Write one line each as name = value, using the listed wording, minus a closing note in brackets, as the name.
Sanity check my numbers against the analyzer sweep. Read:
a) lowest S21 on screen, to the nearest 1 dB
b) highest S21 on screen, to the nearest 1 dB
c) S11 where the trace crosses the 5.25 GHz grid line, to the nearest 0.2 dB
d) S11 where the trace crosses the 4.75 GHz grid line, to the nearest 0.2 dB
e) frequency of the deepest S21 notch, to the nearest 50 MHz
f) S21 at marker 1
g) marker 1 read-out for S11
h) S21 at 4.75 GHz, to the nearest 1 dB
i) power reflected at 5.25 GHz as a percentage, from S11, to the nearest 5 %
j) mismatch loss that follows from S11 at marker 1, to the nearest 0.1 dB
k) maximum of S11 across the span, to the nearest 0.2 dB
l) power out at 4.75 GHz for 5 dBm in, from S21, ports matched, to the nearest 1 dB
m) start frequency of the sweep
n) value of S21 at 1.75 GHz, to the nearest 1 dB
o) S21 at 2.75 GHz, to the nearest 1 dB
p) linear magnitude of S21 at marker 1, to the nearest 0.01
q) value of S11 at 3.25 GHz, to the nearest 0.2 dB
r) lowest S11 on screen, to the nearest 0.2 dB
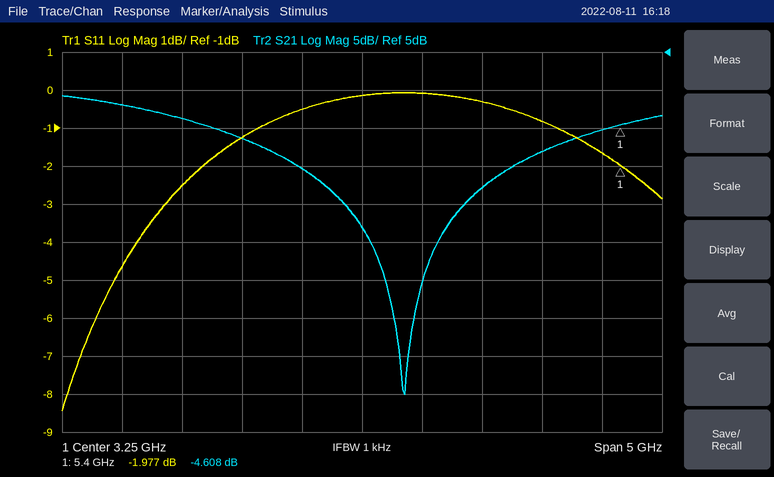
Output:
lowest S21 on screen, to the nearest 1 dB = -40 dB
highest S21 on screen, to the nearest 1 dB = -1 dB
S11 where the trace crosses the 5.25 GHz grid line, to the nearest 0.2 dB = -1.6 dB
S11 where the trace crosses the 4.75 GHz grid line, to the nearest 0.2 dB = -0.8 dB
frequency of the deepest S21 notch, to the nearest 50 MHz = 3.60 GHz
S21 at marker 1 = -4.608 dB
marker 1 read-out for S11 = -1.977 dB
S21 at 4.75 GHz, to the nearest 1 dB = -8 dB
power reflected at 5.25 GHz as a percentage, from S11, to the nearest 5 % = 70 %
mismatch loss that follows from S11 at marker 1, to the nearest 0.1 dB = 4.4 dB
maximum of S11 across the span, to the nearest 0.2 dB = 0.0 dB
power out at 4.75 GHz for 5 dBm in, from S21, ports matched, to the nearest 1 dB = -3 dBm
start frequency of the sweep = 750 MHz
value of S21 at 1.75 GHz, to the nearest 1 dB = -4 dB
S21 at 2.75 GHz, to the nearest 1 dB = -10 dB
linear magnitude of S21 at marker 1, to the nearest 0.01 = 0.59
value of S11 at 3.25 GHz, to the nearest 0.2 dB = -0.2 dB
lowest S11 on screen, to the nearest 0.2 dB = -8.4 dB
